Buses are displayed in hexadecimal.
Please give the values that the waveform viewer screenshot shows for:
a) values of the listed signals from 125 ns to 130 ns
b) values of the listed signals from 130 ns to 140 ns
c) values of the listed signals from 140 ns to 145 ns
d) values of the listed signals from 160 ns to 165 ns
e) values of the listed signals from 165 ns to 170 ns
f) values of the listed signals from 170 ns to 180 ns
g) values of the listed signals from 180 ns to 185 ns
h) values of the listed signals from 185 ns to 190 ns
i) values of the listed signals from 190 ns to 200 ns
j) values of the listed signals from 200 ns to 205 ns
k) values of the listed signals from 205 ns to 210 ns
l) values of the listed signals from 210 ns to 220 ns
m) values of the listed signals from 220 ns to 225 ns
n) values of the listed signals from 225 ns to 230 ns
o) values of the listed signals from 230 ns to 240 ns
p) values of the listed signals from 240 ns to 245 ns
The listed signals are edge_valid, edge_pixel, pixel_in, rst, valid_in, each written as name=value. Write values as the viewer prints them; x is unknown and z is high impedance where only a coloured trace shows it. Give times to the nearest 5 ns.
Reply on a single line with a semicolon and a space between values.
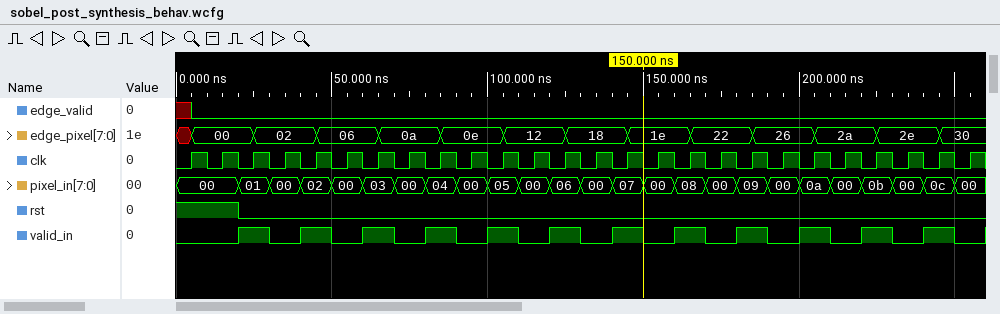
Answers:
edge_valid=0, edge_pixel=18, pixel_in=06, rst=0, valid_in=1; edge_valid=0, edge_pixel=18, pixel_in=00, rst=0, valid_in=0; edge_valid=0, edge_pixel=18, pixel_in=07, rst=0, valid_in=1; edge_valid=0, edge_pixel=1e, pixel_in=08, rst=0, valid_in=1; edge_valid=0, edge_pixel=22, pixel_in=08, rst=0, valid_in=1; edge_valid=0, edge_pixel=22, pixel_in=00, rst=0, valid_in=0; edge_valid=0, edge_pixel=22, pixel_in=09, rst=0, valid_in=1; edge_valid=0, edge_pixel=26, pixel_in=09, rst=0, valid_in=1; edge_valid=0, edge_pixel=26, pixel_in=00, rst=0, valid_in=0; edge_valid=0, edge_pixel=26, pixel_in=0a, rst=0, valid_in=1; edge_valid=0, edge_pixel=2a, pixel_in=0a, rst=0, valid_in=1; edge_valid=0, edge_pixel=2a, pixel_in=00, rst=0, valid_in=0; edge_valid=0, edge_pixel=2a, pixel_in=0b, rst=0, valid_in=1; edge_valid=0, edge_pixel=2e, pixel_in=0b, rst=0, valid_in=1; edge_valid=0, edge_pixel=2e, pixel_in=00, rst=0, valid_in=0; edge_valid=0, edge_pixel=2e, pixel_in=0c, rst=0, valid_in=1
